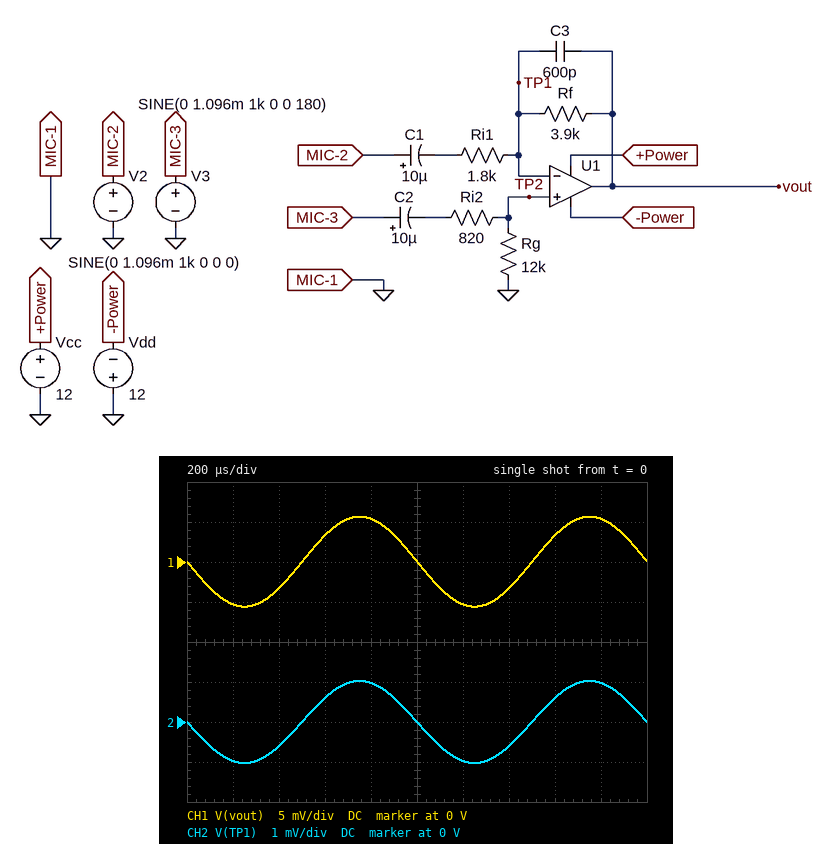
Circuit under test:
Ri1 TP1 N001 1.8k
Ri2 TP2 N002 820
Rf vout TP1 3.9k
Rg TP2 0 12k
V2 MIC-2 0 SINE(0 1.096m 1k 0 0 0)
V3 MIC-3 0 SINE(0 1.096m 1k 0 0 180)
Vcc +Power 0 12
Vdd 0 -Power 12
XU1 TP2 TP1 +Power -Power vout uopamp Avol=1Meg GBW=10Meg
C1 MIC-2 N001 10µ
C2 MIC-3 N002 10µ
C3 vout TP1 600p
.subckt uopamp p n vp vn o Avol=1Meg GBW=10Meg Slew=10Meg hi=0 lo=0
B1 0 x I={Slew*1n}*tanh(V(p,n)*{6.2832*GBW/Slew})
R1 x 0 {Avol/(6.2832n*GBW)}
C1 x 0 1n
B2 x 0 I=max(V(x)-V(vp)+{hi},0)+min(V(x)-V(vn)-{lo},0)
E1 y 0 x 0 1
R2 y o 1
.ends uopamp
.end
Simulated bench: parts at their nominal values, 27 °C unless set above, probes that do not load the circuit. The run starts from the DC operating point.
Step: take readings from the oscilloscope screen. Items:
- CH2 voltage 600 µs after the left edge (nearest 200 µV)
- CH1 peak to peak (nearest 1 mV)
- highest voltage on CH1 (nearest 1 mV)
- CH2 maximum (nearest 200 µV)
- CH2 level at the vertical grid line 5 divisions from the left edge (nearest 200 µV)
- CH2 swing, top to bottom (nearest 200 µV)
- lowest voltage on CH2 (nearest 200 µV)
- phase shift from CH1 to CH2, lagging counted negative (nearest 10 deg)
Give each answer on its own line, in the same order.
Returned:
600 µV
11 mV
6 mV
1.0 mV
0 V
2.0 mV
-1.0 mV
0 deg
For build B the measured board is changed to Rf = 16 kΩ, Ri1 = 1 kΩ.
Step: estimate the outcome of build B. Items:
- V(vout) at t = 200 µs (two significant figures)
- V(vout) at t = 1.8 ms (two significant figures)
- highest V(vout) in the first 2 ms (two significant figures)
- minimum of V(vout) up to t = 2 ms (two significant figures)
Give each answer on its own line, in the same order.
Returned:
-32 mV
34 mV
35 mV
-34 mV
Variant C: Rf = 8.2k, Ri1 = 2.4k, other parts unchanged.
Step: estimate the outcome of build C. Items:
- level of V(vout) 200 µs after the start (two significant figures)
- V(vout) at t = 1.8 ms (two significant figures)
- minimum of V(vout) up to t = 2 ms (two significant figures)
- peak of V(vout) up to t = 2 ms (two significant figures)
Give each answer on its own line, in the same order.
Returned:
-7.8 mV
8.0 mV
-8.2 mV
8.3 mV
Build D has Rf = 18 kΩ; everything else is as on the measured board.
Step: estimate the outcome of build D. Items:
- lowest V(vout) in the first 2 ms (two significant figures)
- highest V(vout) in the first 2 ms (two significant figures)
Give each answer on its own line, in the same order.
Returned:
-22 mV
22 mV
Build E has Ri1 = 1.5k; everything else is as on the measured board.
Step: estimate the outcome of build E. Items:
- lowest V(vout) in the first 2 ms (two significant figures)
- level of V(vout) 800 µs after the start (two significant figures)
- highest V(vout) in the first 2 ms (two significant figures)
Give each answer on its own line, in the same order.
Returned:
-6.5 mV
6.3 mV
6.6 mV
